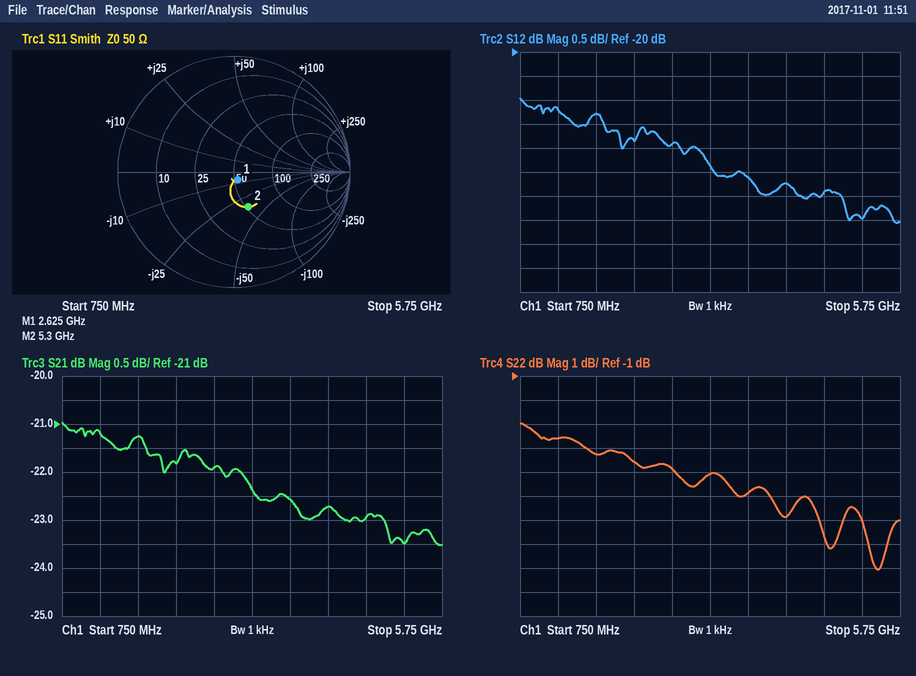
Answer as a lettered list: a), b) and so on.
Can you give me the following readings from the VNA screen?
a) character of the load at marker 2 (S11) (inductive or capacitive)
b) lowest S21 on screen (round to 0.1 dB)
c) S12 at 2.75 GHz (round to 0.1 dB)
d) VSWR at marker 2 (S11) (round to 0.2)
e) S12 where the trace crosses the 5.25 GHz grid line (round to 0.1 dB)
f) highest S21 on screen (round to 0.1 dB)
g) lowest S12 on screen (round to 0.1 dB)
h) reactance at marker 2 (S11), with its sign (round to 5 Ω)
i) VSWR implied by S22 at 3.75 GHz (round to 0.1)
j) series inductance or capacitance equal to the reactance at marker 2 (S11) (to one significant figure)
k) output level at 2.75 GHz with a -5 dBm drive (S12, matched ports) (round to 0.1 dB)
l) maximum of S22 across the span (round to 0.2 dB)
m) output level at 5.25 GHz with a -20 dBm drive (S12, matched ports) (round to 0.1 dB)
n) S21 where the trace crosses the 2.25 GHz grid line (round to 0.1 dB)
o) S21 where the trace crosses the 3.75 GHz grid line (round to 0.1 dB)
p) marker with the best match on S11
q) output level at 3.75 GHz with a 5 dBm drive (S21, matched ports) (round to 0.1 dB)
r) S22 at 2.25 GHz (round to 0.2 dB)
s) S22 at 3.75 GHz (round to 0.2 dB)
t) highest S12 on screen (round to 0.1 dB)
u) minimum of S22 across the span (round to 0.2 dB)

a) capacitive
b) -23.5 dB
c) -21.9 dB
d) 2.0
e) -23.5 dB
f) -21.0 dB
g) -23.6 dB
h) -35 Ω
i) 3.1
j) 900 fF
k) -26.9 dBm
l) -3.0 dB
m) -43.5 dBm
n) -21.8 dB
o) -22.6 dB
p) marker 1
q) -17.6 dBm
r) -4.6 dB
s) -5.8 dB
t) -21.0 dB
u) -9.0 dB
